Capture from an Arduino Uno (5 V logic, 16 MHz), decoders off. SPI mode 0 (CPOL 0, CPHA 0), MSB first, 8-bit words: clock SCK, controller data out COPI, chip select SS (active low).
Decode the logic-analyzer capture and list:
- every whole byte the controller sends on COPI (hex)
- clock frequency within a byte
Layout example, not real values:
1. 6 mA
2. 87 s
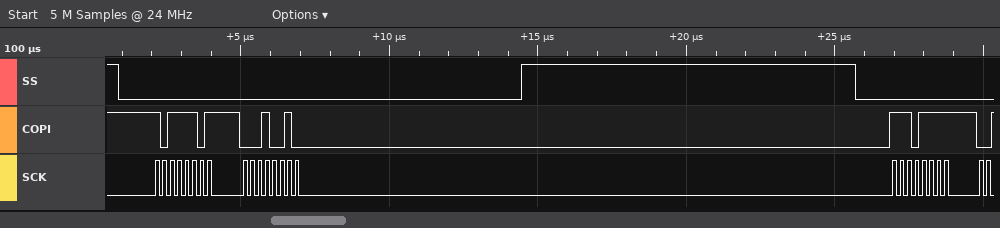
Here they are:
1. BD 12 EF
2. 4 MHz
